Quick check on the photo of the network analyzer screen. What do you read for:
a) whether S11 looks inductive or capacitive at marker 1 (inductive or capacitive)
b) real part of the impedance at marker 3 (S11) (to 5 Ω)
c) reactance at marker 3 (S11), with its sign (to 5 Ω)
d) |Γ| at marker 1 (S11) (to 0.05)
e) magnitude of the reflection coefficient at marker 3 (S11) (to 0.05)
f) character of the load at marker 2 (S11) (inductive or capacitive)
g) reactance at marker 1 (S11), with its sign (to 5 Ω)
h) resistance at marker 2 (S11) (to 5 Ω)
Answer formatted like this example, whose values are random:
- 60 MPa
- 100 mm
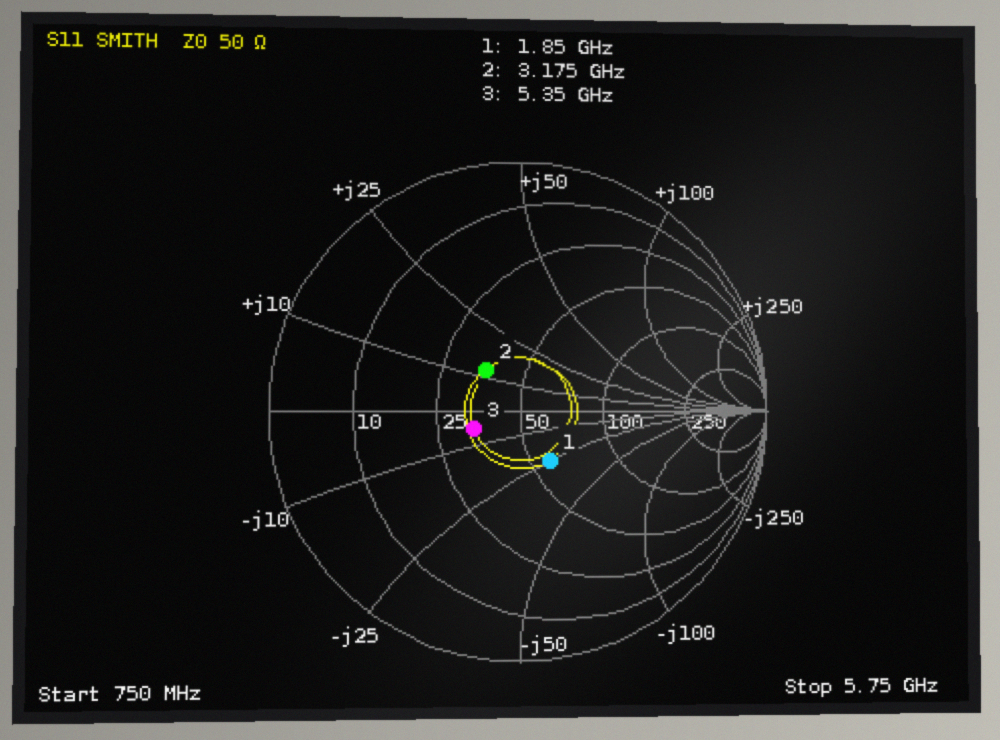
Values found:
- capacitive
- 35 Ω
- -5 Ω
- 0.25
- 0.20
- inductive
- -25 Ω
- 35 Ω
